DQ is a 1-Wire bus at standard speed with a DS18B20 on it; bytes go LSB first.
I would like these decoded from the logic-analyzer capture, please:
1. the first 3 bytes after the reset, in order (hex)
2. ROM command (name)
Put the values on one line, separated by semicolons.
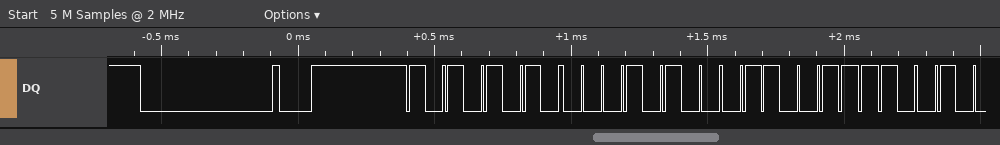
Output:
55 28 E6; Match ROM
